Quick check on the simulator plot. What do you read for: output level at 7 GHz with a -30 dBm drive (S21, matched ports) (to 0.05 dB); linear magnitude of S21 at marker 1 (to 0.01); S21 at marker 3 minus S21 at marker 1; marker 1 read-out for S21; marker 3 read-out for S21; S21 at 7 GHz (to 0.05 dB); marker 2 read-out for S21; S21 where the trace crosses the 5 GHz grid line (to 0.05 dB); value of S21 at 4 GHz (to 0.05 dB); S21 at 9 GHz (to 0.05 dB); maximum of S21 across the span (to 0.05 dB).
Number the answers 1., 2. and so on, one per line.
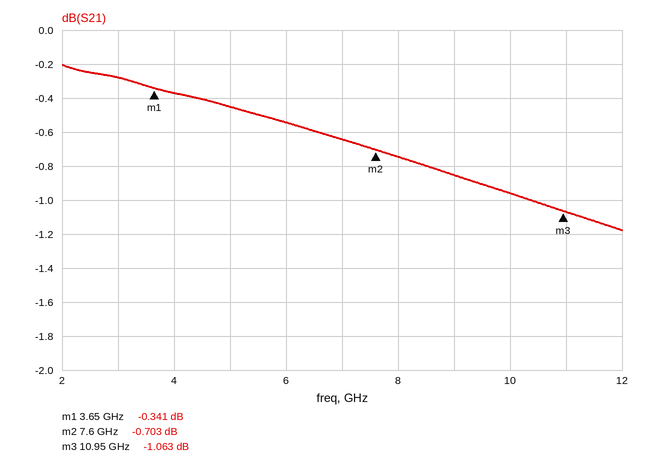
1. -30.65 dBm
2. 0.96
3. -0.722 dB
4. -0.341 dB
5. -1.063 dB
6. -0.65 dB
7. -0.703 dB
8. -0.45 dB
9. -0.35 dB
10. -0.85 dB
11. -0.20 dB
